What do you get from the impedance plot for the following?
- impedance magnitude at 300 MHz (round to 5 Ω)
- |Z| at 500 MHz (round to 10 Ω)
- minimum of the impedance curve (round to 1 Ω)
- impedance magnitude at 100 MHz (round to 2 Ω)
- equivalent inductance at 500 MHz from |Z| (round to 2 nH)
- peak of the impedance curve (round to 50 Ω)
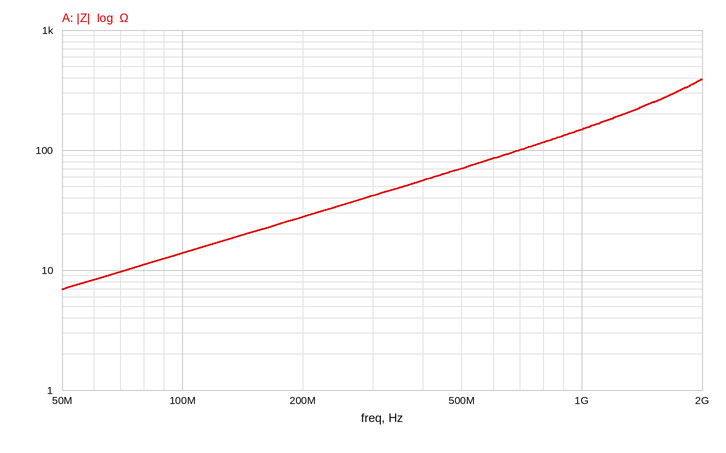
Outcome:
40 Ω
70 Ω
7 Ω
14 Ω
22 nH
400 Ω
